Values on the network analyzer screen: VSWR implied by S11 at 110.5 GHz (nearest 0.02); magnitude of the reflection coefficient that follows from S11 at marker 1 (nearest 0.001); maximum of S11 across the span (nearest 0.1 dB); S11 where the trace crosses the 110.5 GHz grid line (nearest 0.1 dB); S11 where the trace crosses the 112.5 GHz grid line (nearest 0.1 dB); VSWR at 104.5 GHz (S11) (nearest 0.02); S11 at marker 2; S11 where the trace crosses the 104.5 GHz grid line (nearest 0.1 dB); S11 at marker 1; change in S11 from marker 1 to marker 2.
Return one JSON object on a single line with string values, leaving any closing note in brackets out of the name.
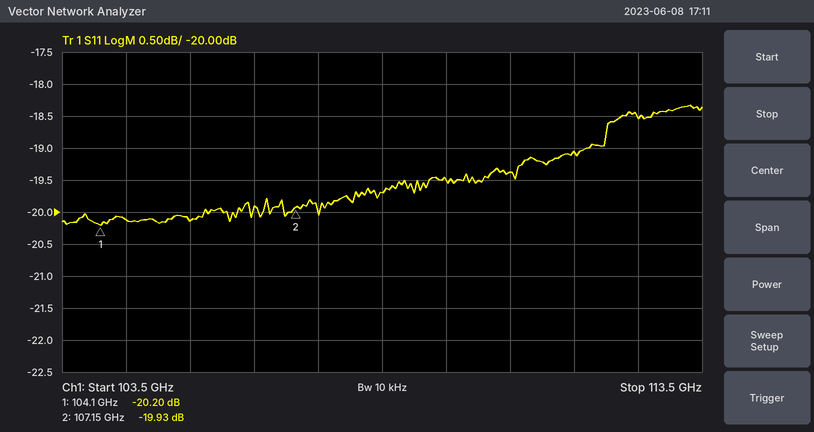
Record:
{"VSWR implied by S11 at 110.5 GHz": "1.24", "magnitude of the reflection coefficient that follows from S11 at marker 1": "0.098", "maximum of S11 across the span": "-18.3 dB", "S11 where the trace crosses the 110.5 GHz grid line": "-19.4 dB", "S11 where the trace crosses the 112.5 GHz grid line": "-18.5 dB", "VSWR at 104.5 GHz (S11)": "1.22", "S11 at marker 2": "-19.93 dB", "S11 where the trace crosses the 104.5 GHz grid line": "-20.1 dB", "S11 at marker 1": "-20.20 dB", "change in S11 from marker 1 to marker 2": "0.27 dB"}
